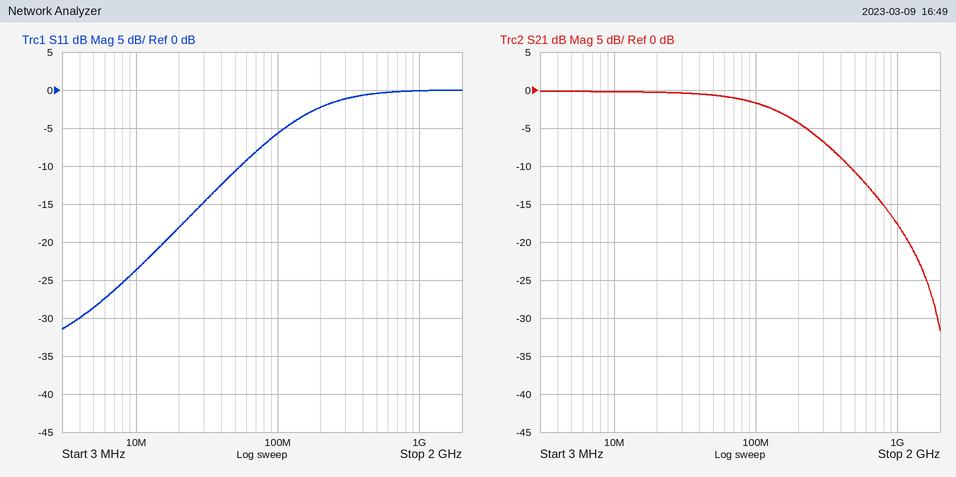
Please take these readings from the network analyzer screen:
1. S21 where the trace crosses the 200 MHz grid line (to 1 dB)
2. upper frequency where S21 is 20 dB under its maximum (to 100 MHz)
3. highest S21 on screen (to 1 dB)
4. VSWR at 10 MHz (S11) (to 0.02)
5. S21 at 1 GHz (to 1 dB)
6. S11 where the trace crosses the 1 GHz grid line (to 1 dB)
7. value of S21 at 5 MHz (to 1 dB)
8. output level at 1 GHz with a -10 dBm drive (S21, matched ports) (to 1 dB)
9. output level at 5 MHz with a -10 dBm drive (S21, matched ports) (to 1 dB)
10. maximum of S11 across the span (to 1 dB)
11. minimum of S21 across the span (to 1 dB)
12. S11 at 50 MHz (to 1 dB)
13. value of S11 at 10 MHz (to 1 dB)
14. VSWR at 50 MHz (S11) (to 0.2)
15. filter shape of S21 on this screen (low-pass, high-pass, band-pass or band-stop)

-4 dB
1.2 GHz
0 dB
1.14
-18 dB
0 dB
0 dB
-28 dBm
-10 dBm
0 dB
-32 dB
-11 dB
-24 dB
1.8
low-pass
